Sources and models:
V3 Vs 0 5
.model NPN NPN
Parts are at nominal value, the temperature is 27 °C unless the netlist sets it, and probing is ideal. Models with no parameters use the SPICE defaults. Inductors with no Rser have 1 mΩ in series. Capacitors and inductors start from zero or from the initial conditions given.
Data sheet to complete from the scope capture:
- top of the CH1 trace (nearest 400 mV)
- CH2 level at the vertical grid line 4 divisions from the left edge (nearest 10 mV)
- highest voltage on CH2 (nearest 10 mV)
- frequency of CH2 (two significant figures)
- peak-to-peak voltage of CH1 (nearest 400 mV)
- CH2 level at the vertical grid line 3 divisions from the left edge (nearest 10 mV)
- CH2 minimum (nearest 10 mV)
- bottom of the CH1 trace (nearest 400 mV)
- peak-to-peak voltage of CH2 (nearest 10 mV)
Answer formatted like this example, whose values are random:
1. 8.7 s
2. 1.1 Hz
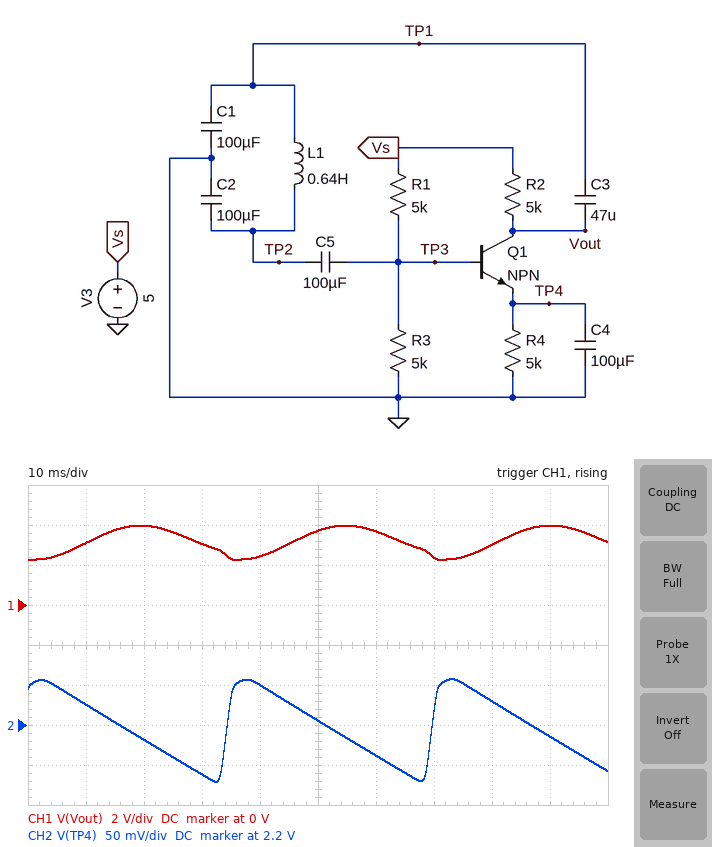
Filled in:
1. 4.0 V
2. 2.25 V
3. 2.26 V
4. 28 Hz
5. 1.6 V
6. 2.14 V
7. 2.13 V
8. 2.4 V
9. 130 mV
